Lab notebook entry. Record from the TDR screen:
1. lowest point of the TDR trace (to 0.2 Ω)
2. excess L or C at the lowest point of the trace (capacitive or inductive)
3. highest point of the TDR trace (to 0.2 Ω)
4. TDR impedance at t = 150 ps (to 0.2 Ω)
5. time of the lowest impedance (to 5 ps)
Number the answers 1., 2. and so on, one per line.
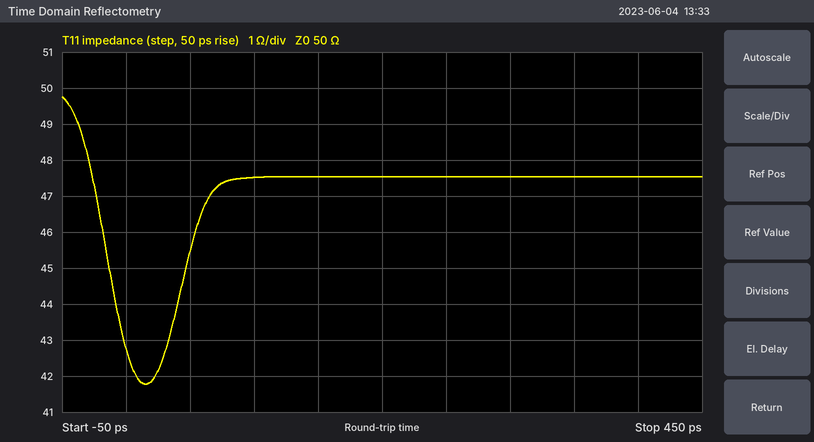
1. 41.8 Ω
2. capacitive
3. 49.8 Ω
4. 47.6 Ω
5. 15 ps
